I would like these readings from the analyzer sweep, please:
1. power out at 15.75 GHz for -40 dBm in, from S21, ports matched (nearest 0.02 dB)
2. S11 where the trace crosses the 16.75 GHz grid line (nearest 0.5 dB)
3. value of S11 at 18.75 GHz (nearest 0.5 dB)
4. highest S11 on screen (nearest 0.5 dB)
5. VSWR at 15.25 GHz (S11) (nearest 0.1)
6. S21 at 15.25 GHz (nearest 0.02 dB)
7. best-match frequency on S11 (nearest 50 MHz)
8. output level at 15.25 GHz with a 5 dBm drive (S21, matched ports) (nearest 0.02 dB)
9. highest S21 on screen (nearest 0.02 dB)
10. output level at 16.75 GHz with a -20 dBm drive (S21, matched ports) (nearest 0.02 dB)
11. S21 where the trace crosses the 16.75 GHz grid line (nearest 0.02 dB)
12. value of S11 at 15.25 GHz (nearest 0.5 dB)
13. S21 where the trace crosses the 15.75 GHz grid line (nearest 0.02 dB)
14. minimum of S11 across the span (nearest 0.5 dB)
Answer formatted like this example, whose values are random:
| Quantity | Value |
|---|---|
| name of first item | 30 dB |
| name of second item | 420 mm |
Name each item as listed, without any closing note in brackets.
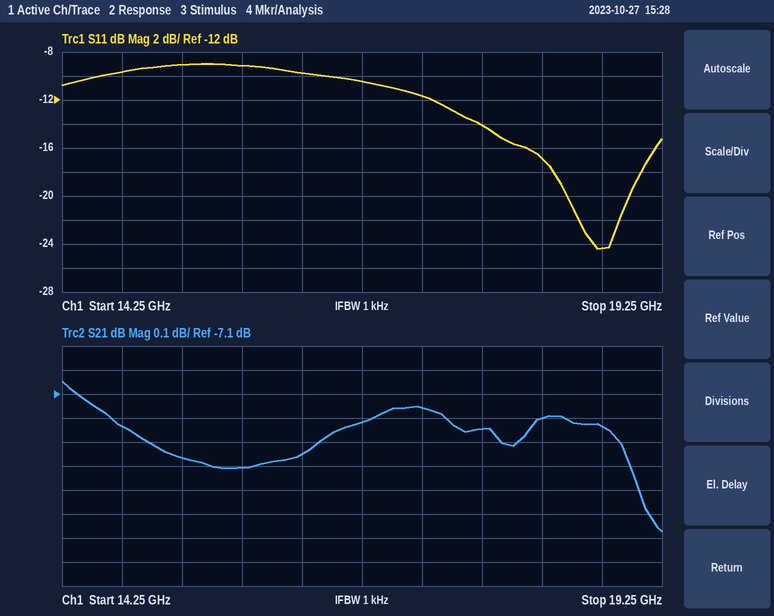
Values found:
| Quantity | Value |
|---|---|
| power out at 15.75 GHz for -40 dBm in, from S21, ports matched | -47.40 dBm |
| S11 where the trace crosses the 16.75 GHz grid line | -10.5 dB |
| value of S11 at 18.75 GHz | -24.5 dB |
| highest S11 on screen | -9.0 dB |
| VSWR at 15.25 GHz (S11) | 2.1 |
| S21 at 15.25 GHz | -7.36 dB |
| best-match frequency on S11 | 18.70 GHz |
| output level at 15.25 GHz with a 5 dBm drive (S21, matched ports) | -2.36 dBm |
| highest S21 on screen | -7.04 dB |
| output level at 16.75 GHz with a -20 dBm drive (S21, matched ports) | -27.22 dBm |
| S21 where the trace crosses the 16.75 GHz grid line | -7.22 dB |
| value of S11 at 15.25 GHz | -9.0 dB |
| S21 where the trace crosses the 15.75 GHz grid line | -7.40 dB |
| minimum of S11 across the span | -24.5 dB |
